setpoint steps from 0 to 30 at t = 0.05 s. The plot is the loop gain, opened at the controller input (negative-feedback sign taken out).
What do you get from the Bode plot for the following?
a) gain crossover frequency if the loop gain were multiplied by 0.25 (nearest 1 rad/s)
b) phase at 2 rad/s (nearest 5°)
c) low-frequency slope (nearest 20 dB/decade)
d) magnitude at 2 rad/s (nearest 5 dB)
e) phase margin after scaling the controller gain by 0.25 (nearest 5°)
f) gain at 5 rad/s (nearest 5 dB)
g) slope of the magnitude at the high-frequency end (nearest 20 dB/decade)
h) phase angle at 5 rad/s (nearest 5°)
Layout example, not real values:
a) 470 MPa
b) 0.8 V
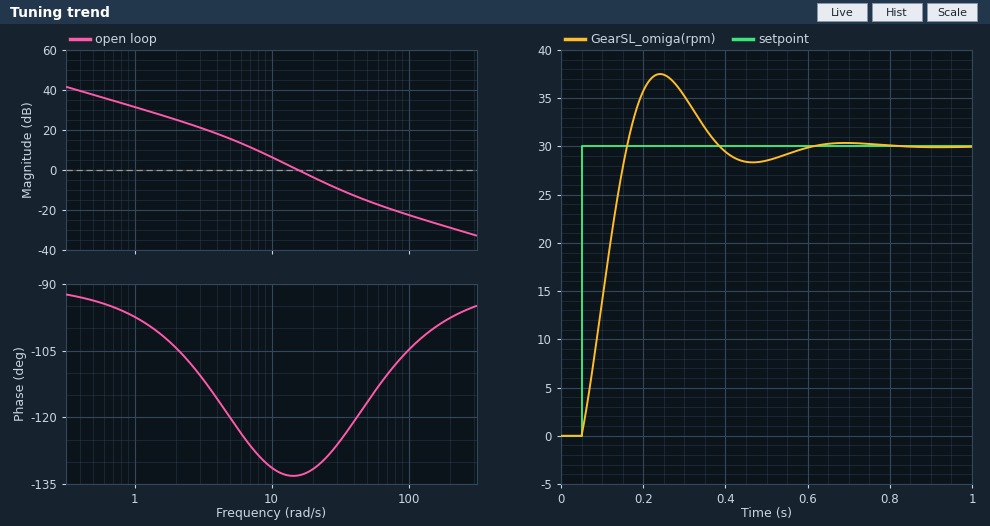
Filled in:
a) 7 rad/s
b) -105°
c) -20 dB/decade
d) 25 dB
e) 55°
f) 15 dB
g) -20 dB/decade
h) -120°
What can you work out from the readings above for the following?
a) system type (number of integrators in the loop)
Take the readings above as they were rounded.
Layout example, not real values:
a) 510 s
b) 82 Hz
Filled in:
a) 1
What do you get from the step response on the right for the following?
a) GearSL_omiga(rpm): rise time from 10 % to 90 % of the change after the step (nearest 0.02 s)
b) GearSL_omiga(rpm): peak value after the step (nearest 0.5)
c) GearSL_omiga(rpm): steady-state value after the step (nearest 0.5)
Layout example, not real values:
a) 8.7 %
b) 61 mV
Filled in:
a) 0.08 s
b) 37.5
c) 30.0
